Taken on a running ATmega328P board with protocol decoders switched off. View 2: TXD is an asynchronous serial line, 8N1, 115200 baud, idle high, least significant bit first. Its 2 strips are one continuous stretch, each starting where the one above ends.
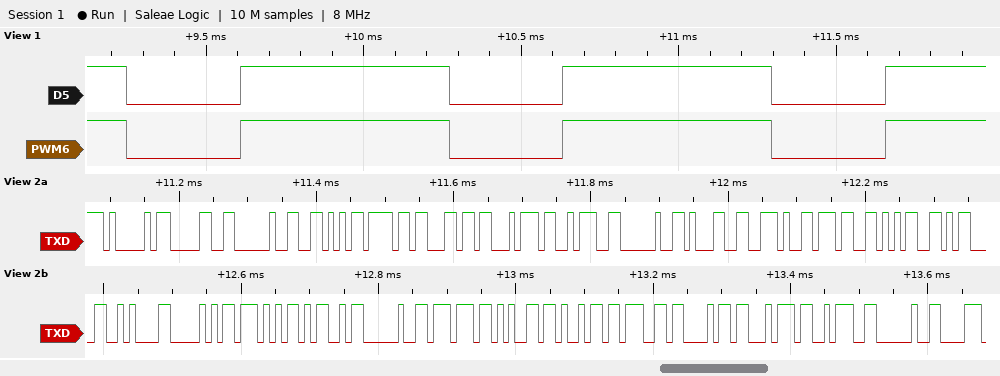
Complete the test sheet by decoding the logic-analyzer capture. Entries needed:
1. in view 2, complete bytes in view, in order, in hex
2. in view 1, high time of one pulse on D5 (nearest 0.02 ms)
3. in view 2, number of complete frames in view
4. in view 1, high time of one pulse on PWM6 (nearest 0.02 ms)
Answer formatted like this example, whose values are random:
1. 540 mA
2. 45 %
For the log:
1. 41 30 20 56 6F 6C 74 3A 20 31 2E 37 35 0D 0A 50 57 4D 20 77 65 69 67 68 74 3A 20
2. 0.66 ms
3. 27
4. 0.66 ms
